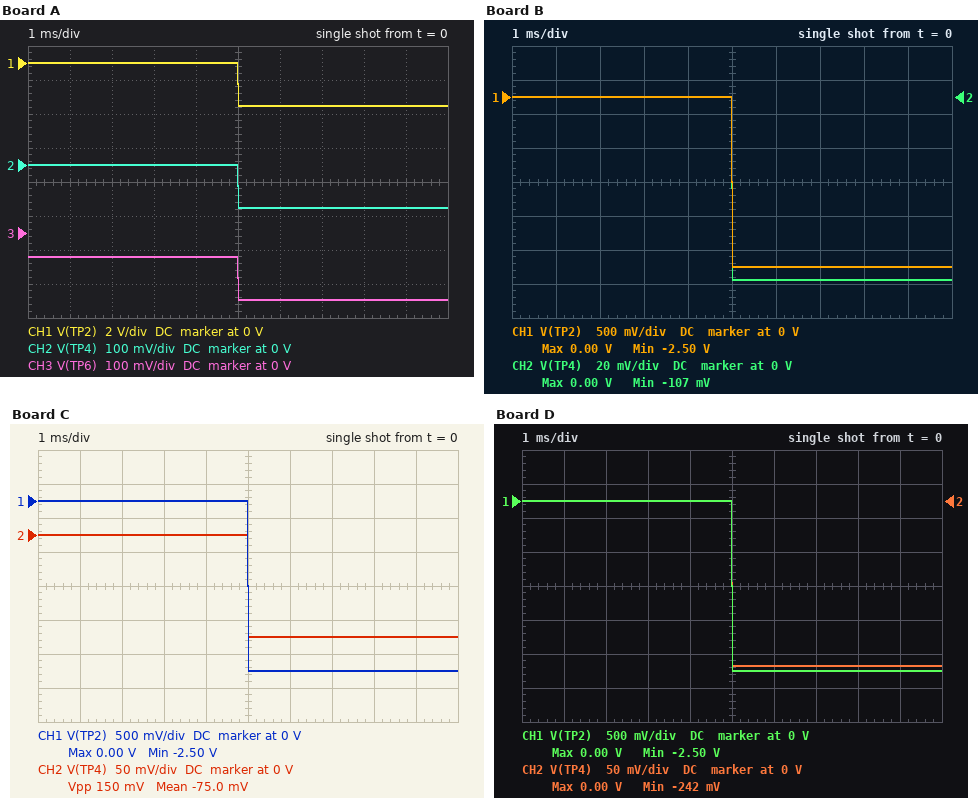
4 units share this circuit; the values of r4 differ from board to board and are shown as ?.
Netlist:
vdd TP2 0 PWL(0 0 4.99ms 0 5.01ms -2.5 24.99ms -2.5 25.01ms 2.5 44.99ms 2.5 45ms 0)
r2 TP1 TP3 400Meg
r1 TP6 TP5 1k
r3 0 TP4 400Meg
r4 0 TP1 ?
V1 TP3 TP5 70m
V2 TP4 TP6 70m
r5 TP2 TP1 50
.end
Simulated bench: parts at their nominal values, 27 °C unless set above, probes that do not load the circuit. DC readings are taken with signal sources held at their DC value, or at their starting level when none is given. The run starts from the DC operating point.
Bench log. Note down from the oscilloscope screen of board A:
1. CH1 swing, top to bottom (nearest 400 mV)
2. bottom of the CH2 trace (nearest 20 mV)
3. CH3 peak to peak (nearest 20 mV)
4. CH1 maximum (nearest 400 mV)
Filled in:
2.4 V
-120 mV
120 mV
0 V
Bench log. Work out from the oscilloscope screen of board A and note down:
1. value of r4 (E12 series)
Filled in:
5.6 Ω
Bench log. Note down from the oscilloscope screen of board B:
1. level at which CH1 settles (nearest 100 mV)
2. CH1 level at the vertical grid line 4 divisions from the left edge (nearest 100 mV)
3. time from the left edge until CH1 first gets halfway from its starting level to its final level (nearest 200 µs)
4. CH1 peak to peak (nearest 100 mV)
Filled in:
-2.5 V
0 V
5.0 ms
2.5 V
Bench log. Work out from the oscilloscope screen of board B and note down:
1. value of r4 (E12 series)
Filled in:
4.7 Ω
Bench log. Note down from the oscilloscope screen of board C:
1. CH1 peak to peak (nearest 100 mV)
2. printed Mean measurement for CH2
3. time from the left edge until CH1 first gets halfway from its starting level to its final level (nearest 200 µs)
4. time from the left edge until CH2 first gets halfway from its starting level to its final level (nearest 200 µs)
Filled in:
2.5 V
-75.0 mV
5.0 ms
5.0 ms
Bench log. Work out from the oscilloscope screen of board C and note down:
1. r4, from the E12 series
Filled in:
6.8 Ω
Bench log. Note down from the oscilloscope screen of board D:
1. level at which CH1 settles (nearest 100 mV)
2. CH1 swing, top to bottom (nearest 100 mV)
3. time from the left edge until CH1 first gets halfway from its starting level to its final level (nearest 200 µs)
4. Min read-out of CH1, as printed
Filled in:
-2.5 V
2.5 V
5.0 ms
-2.50 V
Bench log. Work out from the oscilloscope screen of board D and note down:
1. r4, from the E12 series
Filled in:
12 Ω
